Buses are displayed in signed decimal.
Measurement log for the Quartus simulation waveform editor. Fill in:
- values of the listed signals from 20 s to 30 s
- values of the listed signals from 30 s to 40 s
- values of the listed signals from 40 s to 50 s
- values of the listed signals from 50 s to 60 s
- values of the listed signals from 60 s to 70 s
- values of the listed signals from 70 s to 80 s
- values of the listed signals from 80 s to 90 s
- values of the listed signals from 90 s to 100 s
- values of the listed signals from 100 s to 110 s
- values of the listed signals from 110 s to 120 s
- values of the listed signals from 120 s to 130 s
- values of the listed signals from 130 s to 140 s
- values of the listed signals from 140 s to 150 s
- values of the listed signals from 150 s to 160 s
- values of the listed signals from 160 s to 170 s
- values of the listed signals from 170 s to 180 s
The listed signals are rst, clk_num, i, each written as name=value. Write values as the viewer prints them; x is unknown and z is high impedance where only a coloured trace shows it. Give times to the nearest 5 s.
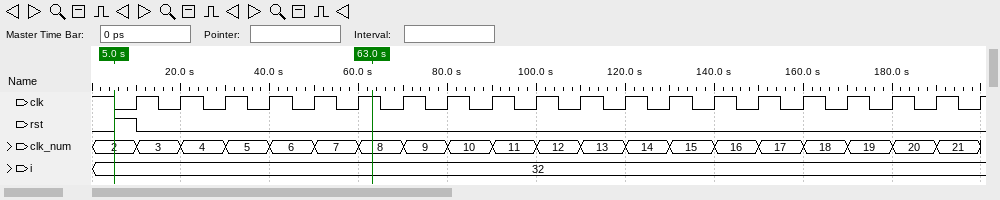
rst=0, clk_num=4, i=32
rst=0, clk_num=5, i=32
rst=0, clk_num=6, i=32
rst=0, clk_num=7, i=32
rst=0, clk_num=8, i=32
rst=0, clk_num=9, i=32
rst=0, clk_num=10, i=32
rst=0, clk_num=11, i=32
rst=0, clk_num=12, i=32
rst=0, clk_num=13, i=32
rst=0, clk_num=14, i=32
rst=0, clk_num=15, i=32
rst=0, clk_num=16, i=32
rst=0, clk_num=17, i=32
rst=0, clk_num=18, i=32
rst=0, clk_num=19, i=32
